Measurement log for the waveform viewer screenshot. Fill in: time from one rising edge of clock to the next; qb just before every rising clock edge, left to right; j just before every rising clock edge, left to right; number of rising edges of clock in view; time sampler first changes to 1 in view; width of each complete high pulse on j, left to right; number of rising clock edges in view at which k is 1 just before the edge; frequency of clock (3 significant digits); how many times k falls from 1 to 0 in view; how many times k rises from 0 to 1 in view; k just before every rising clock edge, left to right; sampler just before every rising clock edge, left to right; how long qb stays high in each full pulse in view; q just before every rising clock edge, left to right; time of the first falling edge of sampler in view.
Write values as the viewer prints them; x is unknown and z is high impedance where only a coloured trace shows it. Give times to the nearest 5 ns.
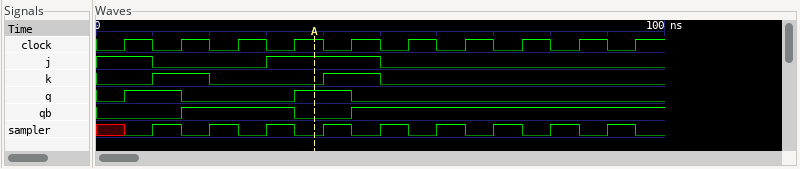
10 ns
0 0 1 1 0 1 1 1 1 1
1 0 0 1 1 0 0 0 0 0
10
10 ns
20 ns
2
100 MHz
2
2
0 1 0 0 1 0 0 0 0 0
x 1 1 1 1 1 1 1 1 1
20 ns
0 1 0 0 1 0 0 0 0 0
15 ns
